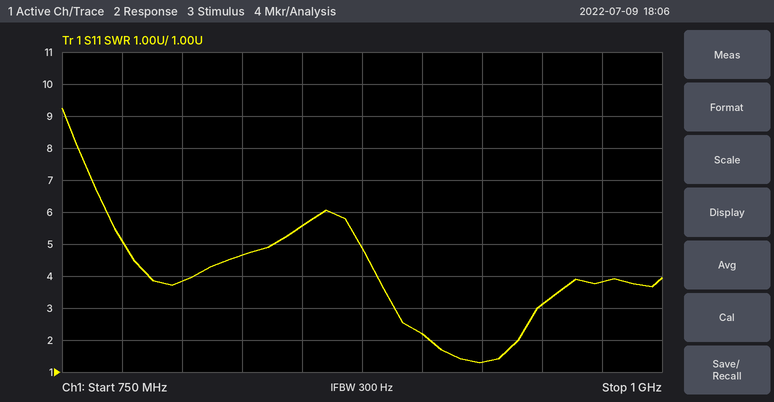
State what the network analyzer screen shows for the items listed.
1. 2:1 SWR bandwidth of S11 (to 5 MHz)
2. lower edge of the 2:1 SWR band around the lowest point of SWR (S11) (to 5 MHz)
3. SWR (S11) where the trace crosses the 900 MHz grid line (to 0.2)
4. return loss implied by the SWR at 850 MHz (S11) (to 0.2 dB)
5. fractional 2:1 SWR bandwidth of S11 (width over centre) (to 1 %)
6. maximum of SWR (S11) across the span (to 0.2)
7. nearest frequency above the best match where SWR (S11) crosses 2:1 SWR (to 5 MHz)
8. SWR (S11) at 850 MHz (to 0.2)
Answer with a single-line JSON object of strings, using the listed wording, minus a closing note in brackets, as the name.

{"2:1 SWR bandwidth of S11": "35 MHz", "lower edge of the 2:1 SWR band around the lowest point of SWR (S11)": "905 MHz", "SWR (S11) where the trace crosses the 900 MHz grid line": "2.2", "return loss implied by the SWR at 850 MHz (S11)": "3.2 dB", "fractional 2:1 SWR bandwidth of S11 (width over centre)": "4 %", "maximum of SWR (S11) across the span": "9.2", "nearest frequency above the best match where SWR (S11) crosses 2:1 SWR": "940 MHz", "SWR (S11) at 850 MHz": "5.6"}
